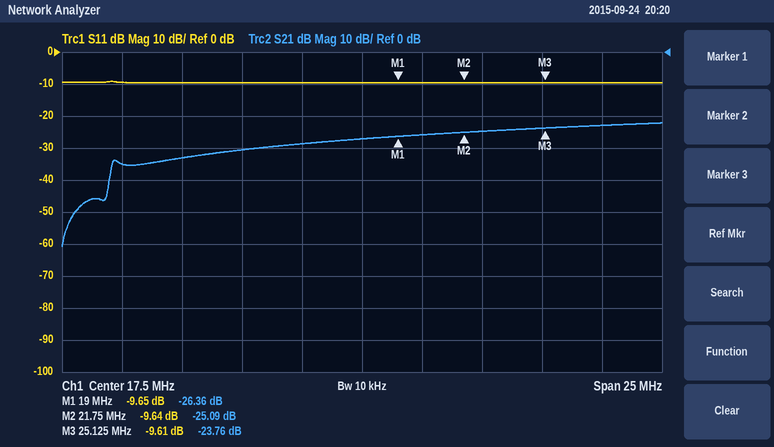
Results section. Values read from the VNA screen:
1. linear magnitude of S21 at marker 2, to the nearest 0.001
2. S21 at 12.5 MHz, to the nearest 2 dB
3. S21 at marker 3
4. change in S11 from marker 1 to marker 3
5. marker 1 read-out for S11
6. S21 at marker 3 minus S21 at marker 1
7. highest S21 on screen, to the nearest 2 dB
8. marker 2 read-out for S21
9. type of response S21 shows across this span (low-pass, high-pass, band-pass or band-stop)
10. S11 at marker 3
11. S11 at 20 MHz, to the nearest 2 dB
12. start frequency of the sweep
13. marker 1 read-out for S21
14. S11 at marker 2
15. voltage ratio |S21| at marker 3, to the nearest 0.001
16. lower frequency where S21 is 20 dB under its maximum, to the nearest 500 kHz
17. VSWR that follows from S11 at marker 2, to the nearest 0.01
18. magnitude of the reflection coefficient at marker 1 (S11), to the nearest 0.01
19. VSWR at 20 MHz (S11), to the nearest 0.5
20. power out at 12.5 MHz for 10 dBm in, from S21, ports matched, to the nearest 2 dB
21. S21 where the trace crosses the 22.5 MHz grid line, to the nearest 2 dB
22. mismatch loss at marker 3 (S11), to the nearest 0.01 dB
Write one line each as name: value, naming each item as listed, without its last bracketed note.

linear magnitude of S21 at marker 2, to the nearest 0.001: 0.056
S21 at 12.5 MHz, to the nearest 2 dB: -30 dB
S21 at marker 3: -23.76 dB
change in S11 from marker 1 to marker 3: 0.04 dB
marker 1 read-out for S11: -9.65 dB
S21 at marker 3 minus S21 at marker 1: 2.60 dB
highest S21 on screen, to the nearest 2 dB: -22 dB
marker 2 read-out for S21: -25.09 dB
type of response S21 shows across this span: high-pass
S11 at marker 3: -9.61 dB
S11 at 20 MHz, to the nearest 2 dB: -10 dB
start frequency of the sweep: 5 MHz
marker 1 read-out for S21: -26.36 dB
S11 at marker 2: -9.64 dB
voltage ratio |S21| at marker 3, to the nearest 0.001: 0.065
lower frequency where S21 is 20 dB under its maximum, to the nearest 500 kHz: 7.0 MHz
VSWR that follows from S11 at marker 2, to the nearest 0.01: 1.98
magnitude of the reflection coefficient at marker 1 (S11), to the nearest 0.01: 0.33
VSWR at 20 MHz (S11), to the nearest 0.5: 2.0
power out at 12.5 MHz for 10 dBm in, from S21, ports matched, to the nearest 2 dB: -20 dBm
S21 where the trace crosses the 22.5 MHz grid line, to the nearest 2 dB: -24 dB
mismatch loss at marker 3 (S11), to the nearest 0.01 dB: 0.50 dB
